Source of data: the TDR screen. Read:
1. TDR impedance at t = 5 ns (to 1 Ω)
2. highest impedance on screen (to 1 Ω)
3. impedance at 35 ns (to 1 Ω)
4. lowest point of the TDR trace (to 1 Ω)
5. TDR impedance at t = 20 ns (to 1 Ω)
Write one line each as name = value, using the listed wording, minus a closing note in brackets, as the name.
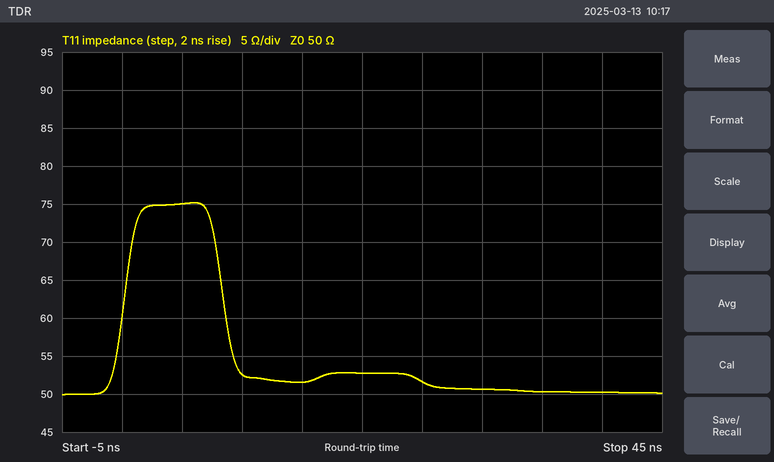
TDR impedance at t = 5 ns = 75 Ω
highest impedance on screen = 75 Ω
impedance at 35 ns = 50 Ω
lowest point of the TDR trace = 50 Ω
TDR impedance at t = 20 ns = 53 Ω
